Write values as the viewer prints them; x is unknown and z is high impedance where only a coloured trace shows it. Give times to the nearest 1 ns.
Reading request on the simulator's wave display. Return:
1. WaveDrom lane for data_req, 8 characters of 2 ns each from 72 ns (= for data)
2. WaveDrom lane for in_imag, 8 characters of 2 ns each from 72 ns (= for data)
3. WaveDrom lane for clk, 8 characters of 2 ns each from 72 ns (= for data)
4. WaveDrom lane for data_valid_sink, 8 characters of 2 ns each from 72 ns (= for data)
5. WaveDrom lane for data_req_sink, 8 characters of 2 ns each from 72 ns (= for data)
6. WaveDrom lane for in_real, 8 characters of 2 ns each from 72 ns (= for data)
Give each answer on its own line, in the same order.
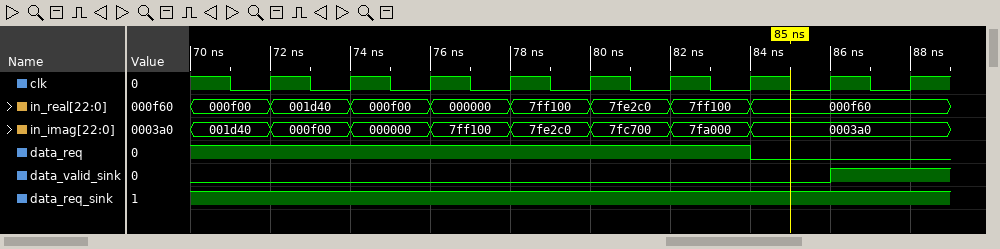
{name: 'data_req', wave: '1.....0.'}
{name: 'in_imag', wave: '=======.', data: '000f00 000000 7ff100 7fe2c0 7fc700 7fa000 0003a0'}
{name: 'clk', wave: 'p.......'}
{name: 'data_valid_sink', wave: '0......1'}
{name: 'data_req_sink', wave: '1.......'}
{name: 'in_real', wave: '=======.', data: '001d40 000f00 000000 7ff100 7fe2c0 7ff100 000f60'}
